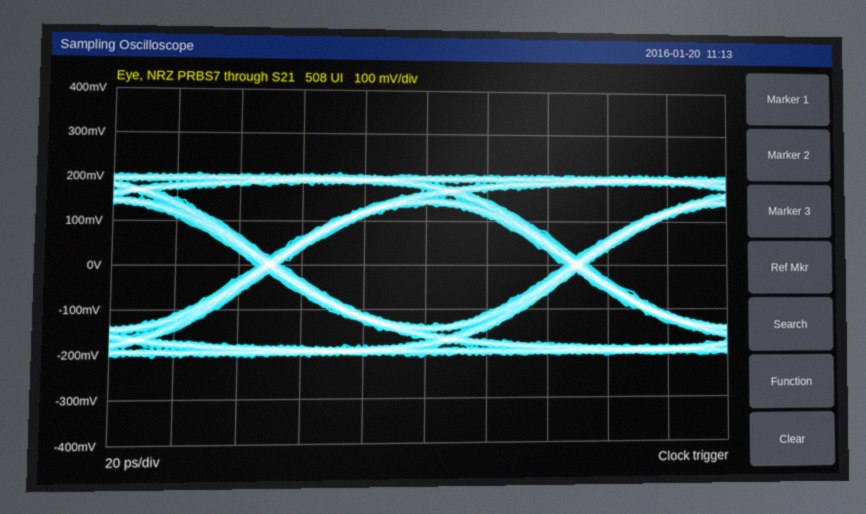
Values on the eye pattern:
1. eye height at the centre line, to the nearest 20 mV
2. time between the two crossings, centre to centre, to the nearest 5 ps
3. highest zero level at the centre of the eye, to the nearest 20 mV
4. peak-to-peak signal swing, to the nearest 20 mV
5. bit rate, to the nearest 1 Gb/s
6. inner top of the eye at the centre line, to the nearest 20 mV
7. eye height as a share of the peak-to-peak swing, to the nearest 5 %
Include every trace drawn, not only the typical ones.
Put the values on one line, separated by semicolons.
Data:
280 mV; 100 ps; -140 mV; 420 mV; 10 Gb/s; 140 mV; 65 %
